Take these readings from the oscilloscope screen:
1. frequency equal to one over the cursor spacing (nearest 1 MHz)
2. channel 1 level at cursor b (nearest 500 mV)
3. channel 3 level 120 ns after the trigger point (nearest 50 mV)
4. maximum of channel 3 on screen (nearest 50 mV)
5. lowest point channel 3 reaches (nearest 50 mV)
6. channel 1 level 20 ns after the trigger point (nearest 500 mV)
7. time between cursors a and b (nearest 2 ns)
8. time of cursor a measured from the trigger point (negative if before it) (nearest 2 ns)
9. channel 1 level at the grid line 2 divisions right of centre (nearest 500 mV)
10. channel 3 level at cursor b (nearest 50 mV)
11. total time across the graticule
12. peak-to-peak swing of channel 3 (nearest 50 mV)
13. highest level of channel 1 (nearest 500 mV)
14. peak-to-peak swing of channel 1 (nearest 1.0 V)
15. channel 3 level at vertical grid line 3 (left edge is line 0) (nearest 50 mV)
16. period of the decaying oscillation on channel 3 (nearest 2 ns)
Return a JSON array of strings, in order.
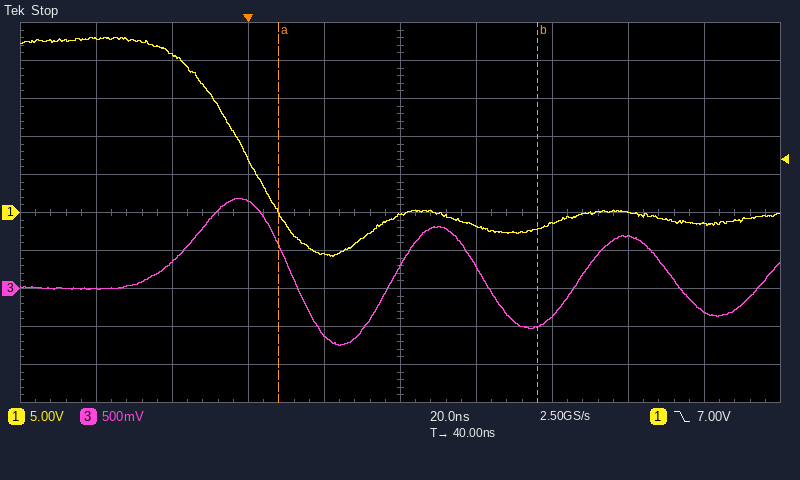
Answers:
["15 MHz", "-2.0 V", "-300 mV", "1.20 V", "-750 mV", "-5.5 V", "68 ns", "+8 ns", "-1.5 V", "-500 mV", "200 ns", "1.95 V", "23.0 V", "29.0 V", "1.15 V", "52 ns"]
